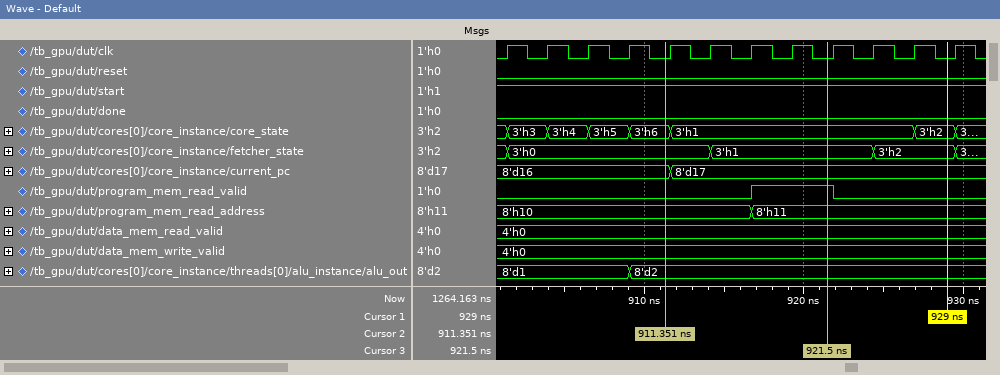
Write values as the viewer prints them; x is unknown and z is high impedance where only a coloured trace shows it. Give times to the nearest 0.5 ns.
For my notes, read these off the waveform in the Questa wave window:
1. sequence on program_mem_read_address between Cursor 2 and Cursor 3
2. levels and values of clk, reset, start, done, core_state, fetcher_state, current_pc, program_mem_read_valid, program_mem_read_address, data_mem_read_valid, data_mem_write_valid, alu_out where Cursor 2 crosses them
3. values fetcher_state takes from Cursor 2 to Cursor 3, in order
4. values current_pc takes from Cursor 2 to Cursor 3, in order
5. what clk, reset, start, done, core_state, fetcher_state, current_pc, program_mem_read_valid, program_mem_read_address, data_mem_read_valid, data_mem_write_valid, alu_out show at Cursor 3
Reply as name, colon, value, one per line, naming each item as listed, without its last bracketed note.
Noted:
sequence on program_mem_read_address between Cursor 2 and Cursor 3: 8'h10, 8'h11
levels and values of clk, reset, start, done, core_state, fetcher_state, current_pc, program_mem_read_valid, program_mem_read_address, data_mem_read_valid, data_mem_write_valid, alu_out where Cursor 2 crosses them: clk=0, reset=0, start=1, done=0, core_state=3'h6, fetcher_state=3'h0, current_pc=8'd16, program_mem_read_valid=0, program_mem_read_address=8'h10, data_mem_read_valid=4'h0, data_mem_write_valid=4'h0, alu_out=8'd2
values fetcher_state takes from Cursor 2 to Cursor 3, in order: 3'h0, 3'h1
values current_pc takes from Cursor 2 to Cursor 3, in order: 8'd16, 8'd17
what clk, reset, start, done, core_state, fetcher_state, current_pc, program_mem_read_valid, program_mem_read_address, data_mem_read_valid, data_mem_write_valid, alu_out show at Cursor 3: clk=0, reset=0, start=1, done=0, core_state=3'h1, fetcher_state=3'h1, current_pc=8'd17, program_mem_read_valid=1, program_mem_read_address=8'h11, data_mem_read_valid=4'h0, data_mem_write_valid=4'h0, alu_out=8'd2
